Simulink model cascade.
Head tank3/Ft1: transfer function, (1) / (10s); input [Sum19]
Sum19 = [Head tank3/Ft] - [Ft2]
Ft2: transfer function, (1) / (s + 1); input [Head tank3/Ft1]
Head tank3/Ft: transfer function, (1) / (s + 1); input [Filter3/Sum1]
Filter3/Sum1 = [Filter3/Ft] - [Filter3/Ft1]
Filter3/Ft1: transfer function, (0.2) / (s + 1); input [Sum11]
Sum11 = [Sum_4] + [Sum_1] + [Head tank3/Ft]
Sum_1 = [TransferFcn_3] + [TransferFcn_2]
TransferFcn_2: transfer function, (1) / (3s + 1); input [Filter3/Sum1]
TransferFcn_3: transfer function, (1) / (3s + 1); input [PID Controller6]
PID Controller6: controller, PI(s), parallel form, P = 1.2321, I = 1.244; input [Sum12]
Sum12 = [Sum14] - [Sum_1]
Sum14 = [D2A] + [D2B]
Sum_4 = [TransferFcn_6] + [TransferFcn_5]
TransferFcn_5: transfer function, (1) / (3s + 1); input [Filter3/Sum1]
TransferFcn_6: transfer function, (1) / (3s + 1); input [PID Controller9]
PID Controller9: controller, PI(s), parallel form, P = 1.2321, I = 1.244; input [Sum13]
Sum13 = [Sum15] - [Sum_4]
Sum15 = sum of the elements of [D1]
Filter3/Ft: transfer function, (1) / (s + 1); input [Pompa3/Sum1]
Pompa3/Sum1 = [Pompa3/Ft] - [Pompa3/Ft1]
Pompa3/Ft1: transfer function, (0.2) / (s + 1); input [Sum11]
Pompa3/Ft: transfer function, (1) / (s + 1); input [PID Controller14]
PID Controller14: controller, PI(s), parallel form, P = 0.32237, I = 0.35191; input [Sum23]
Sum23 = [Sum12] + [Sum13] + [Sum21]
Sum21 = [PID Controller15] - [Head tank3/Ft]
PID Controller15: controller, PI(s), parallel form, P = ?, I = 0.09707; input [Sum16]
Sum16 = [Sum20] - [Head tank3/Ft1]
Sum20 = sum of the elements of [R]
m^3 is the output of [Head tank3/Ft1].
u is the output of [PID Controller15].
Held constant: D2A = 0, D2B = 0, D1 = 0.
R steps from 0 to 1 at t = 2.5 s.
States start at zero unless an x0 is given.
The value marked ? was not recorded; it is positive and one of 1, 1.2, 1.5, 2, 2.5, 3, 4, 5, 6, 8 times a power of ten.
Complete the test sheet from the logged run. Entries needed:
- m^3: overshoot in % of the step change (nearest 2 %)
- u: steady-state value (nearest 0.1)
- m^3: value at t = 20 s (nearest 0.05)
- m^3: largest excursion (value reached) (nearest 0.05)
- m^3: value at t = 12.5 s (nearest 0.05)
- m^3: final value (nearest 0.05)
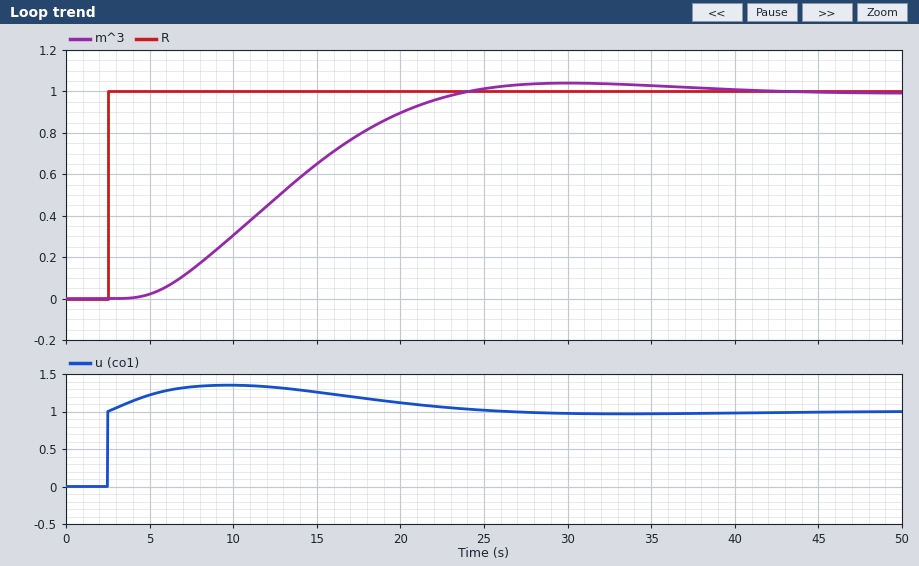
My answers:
4 %
1.0
0.90
1.05
0.50
1.00
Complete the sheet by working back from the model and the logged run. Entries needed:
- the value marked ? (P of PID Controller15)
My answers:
1
